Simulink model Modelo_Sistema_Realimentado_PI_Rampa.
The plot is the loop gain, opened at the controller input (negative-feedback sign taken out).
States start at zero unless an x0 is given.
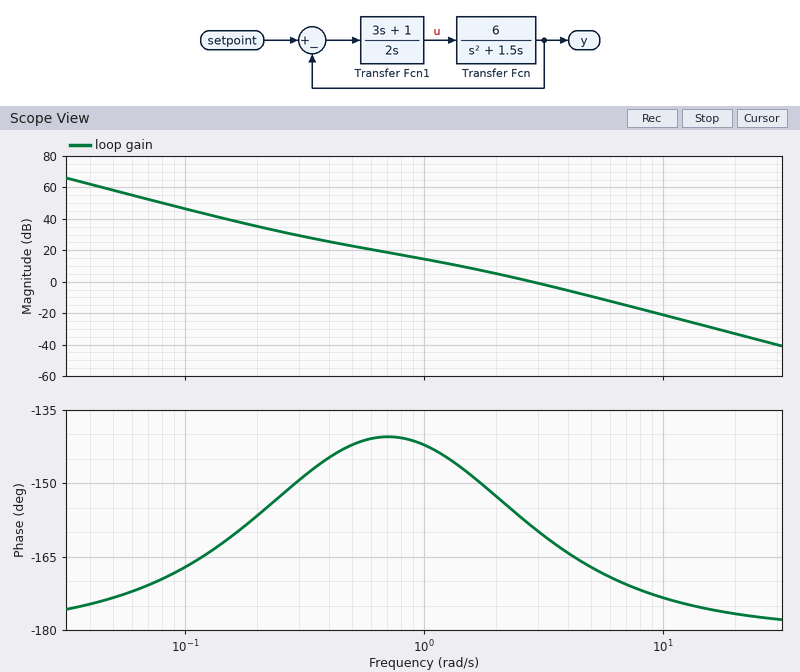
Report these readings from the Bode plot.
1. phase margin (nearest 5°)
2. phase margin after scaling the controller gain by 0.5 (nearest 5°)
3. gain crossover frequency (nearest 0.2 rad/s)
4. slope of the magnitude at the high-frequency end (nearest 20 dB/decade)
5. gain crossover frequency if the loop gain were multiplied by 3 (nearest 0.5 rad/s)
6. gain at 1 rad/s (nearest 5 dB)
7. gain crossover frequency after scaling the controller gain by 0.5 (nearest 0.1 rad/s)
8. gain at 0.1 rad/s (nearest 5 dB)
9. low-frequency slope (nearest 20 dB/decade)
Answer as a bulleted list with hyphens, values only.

- 20°
- 30°
- 2.8 rad/s
- -40 dB/decade
- 5.0 rad/s
- 15 dB
- 1.9 rad/s
- 45 dB
- -40 dB/decade
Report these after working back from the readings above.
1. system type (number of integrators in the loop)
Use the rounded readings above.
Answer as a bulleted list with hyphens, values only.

- 2
